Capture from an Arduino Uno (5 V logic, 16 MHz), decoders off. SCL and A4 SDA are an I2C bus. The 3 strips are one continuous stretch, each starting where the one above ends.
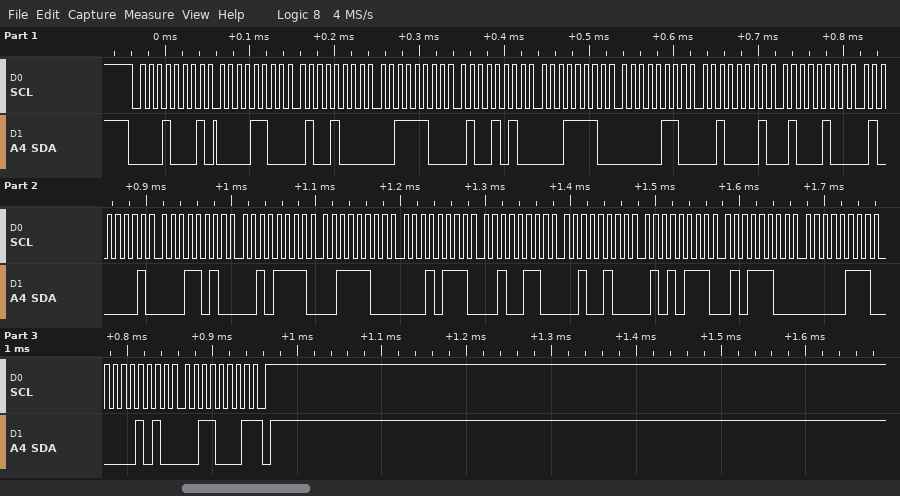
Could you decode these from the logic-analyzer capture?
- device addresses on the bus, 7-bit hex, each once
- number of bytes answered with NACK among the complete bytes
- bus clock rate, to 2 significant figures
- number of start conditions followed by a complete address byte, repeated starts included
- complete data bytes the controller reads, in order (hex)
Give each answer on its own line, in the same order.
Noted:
0x08
1
100 kHz
1
0C 48 3C 4A 1E 06 21 44 41 1A 2F 3C 17 26 24 57 5C 07 0A 31
